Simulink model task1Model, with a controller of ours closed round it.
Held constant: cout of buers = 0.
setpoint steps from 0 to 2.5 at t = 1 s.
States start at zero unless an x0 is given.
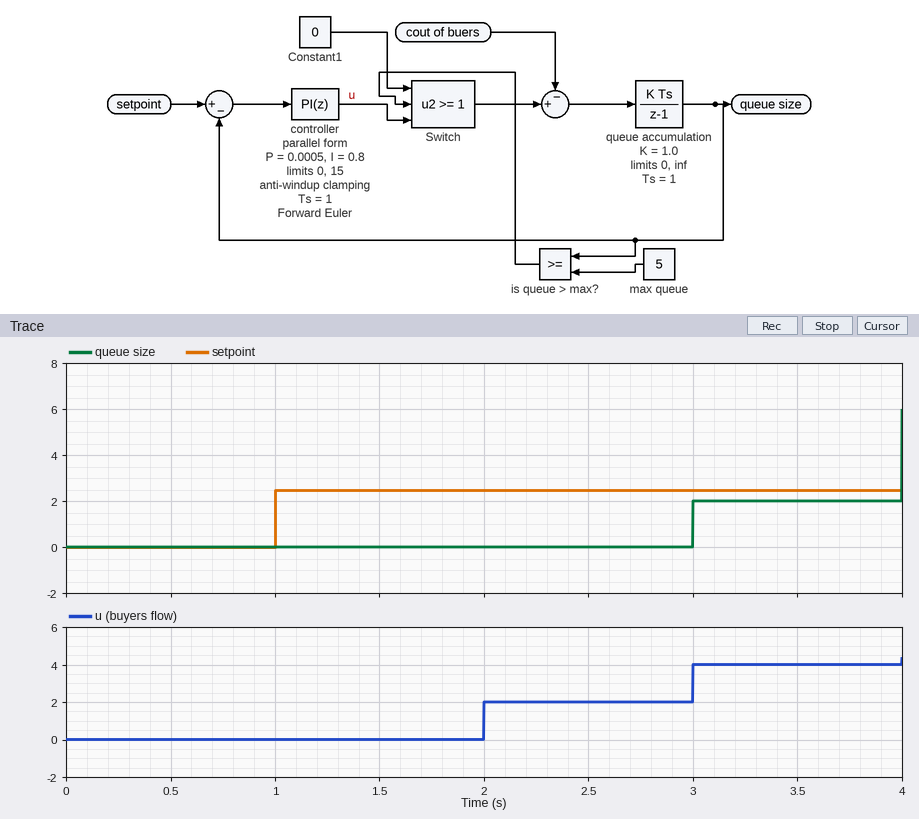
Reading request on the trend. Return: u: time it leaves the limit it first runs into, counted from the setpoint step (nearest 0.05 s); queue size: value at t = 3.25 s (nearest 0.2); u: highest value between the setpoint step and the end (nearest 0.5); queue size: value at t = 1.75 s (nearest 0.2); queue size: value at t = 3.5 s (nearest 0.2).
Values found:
1.00 s
2.0
4.0
0.0
2.0
